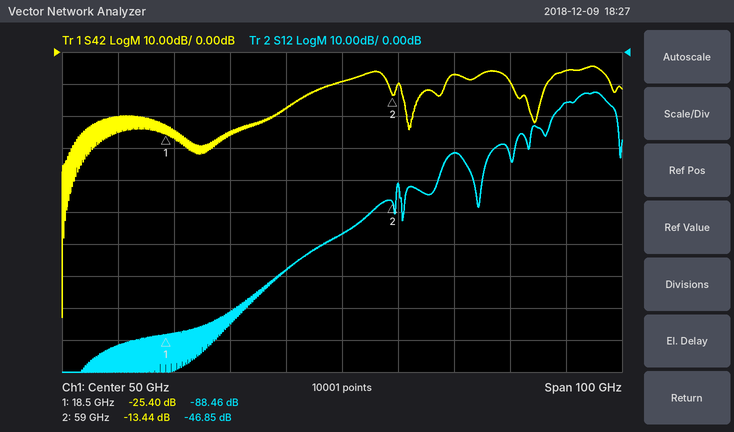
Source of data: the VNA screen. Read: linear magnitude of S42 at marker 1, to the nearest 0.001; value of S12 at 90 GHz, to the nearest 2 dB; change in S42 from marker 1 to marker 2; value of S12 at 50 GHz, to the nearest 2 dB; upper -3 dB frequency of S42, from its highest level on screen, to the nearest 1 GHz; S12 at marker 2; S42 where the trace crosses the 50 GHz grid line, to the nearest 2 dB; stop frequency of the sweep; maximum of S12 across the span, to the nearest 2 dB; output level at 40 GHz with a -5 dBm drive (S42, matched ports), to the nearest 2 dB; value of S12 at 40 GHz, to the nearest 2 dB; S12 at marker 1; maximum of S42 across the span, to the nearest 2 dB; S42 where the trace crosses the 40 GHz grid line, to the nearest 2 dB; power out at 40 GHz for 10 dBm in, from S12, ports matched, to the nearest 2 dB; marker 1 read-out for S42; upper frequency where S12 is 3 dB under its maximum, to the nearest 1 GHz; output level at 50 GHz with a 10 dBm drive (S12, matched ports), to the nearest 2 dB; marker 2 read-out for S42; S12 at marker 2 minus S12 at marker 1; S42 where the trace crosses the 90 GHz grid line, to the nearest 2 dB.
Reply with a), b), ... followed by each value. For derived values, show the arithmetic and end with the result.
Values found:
a) 10^(-25.4/20) ≈ 0.054
b) -16 dB
c) -13.44 − (-25.4) = 11.96 dB
d) -56 dB
e) 97 GHz
f) -46.85 dB
g) -10 dB
h) 100 GHz
i) -12 dB
j) -5 dBm + (-18 dB) = -22 dBm
k) -68 dB
l) -88.46 dB
m) -4 dB
n) -18 dB
o) 10 dBm + (-68 dB) = -58 dBm
p) -25.40 dB
q) 97 GHz
r) 10 dBm + (-56 dB) = -46 dBm
s) -13.44 dB
t) -46.85 − (-88.46) = 41.61 dB
u) -6 dB
